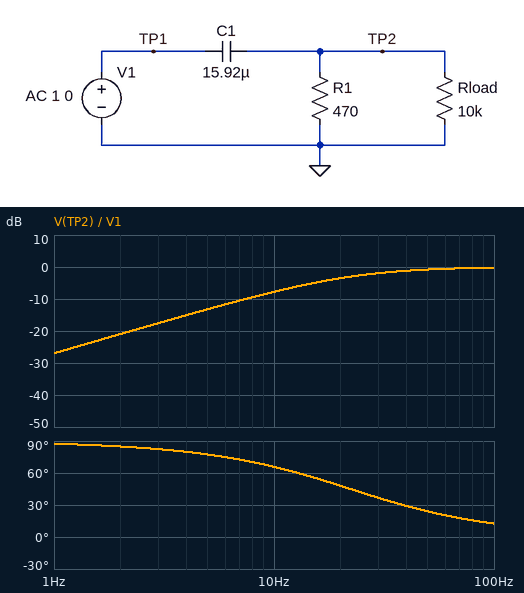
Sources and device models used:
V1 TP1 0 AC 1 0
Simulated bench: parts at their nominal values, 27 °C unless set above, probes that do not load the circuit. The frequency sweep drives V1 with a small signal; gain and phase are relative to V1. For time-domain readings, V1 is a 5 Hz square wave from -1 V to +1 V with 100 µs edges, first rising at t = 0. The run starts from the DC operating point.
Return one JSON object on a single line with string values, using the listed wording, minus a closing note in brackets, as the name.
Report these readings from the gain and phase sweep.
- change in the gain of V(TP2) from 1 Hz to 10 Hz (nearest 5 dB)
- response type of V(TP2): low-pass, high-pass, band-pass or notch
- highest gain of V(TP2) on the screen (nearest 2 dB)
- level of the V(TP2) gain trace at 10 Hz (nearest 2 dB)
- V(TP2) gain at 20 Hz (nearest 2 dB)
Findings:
{"change in the gain of V(TP2) from 1 Hz to 10 Hz": "20 dB", "response type of V(TP2): low-pass, high-pass, band-pass or notch": "high-pass", "highest gain of V(TP2) on the screen": "0 dB", "level of the V(TP2) gain trace at 10 Hz": "-8 dB", "V(TP2) gain at 20 Hz": "-4 dB"}
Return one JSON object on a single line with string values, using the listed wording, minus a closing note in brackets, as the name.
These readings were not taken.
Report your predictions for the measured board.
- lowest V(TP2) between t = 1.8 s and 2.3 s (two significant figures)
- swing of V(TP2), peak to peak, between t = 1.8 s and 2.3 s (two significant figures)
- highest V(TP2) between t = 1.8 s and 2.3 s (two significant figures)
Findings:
{"lowest V(TP2) between t = 1.8 s and 2.3 s": "-2.0 V", "swing of V(TP2), peak to peak, between t = 1.8 s and 2.3 s": "4.0 V", "highest V(TP2) between t = 1.8 s and 2.3 s": "2.0 V"}
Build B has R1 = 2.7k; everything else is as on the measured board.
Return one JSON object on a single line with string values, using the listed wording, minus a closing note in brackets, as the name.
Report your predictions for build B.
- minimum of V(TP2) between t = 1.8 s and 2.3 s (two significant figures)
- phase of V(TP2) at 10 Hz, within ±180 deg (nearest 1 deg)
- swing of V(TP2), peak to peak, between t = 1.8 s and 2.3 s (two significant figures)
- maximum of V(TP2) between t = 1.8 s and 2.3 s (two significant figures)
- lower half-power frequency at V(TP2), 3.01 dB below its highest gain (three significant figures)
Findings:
{"minimum of V(TP2) between t = 1.8 s and 2.3 s": "-1.9 V", "phase of V(TP2) at 10 Hz, within ±180 deg": "25 deg", "swing of V(TP2), peak to peak, between t = 1.8 s and 2.3 s": "3.8 V", "maximum of V(TP2) between t = 1.8 s and 2.3 s": "1.9 V", "lower half-power frequency at V(TP2), 3.01 dB below its highest gain": "4.70 Hz"}
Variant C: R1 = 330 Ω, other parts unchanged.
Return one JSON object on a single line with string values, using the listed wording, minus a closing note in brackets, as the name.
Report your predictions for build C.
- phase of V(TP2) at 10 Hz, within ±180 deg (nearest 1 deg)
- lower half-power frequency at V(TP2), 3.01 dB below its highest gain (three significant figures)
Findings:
{"phase of V(TP2) at 10 Hz, within ±180 deg": "72 deg", "lower half-power frequency at V(TP2), 3.01 dB below its highest gain": "31.3 Hz"}
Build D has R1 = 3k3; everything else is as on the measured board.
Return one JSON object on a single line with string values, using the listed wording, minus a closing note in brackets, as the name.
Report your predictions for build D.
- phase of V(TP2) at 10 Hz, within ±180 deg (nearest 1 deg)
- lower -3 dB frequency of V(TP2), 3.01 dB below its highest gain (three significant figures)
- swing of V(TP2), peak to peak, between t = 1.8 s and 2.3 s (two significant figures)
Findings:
{"phase of V(TP2) at 10 Hz, within ±180 deg": "22 deg", "lower -3 dB frequency of V(TP2), 3.01 dB below its highest gain": "4.03 Hz", "swing of V(TP2), peak to peak, between t = 1.8 s and 2.3 s": "3.7 V"}
